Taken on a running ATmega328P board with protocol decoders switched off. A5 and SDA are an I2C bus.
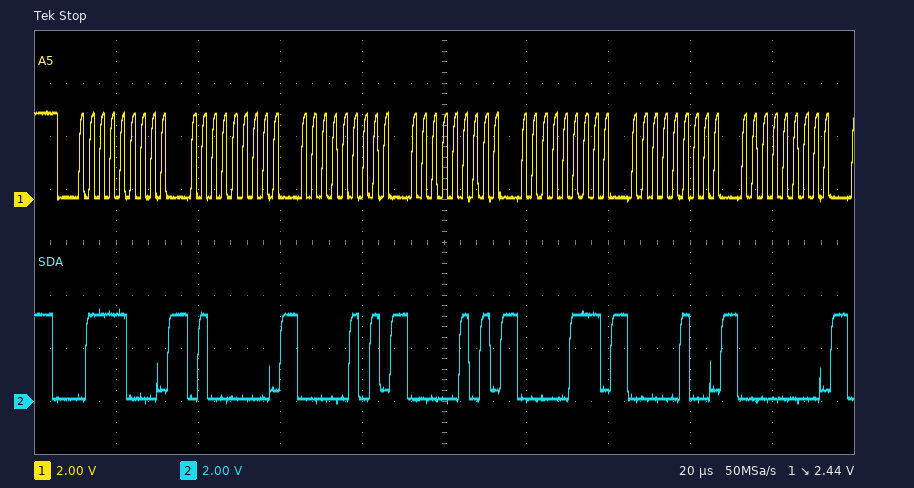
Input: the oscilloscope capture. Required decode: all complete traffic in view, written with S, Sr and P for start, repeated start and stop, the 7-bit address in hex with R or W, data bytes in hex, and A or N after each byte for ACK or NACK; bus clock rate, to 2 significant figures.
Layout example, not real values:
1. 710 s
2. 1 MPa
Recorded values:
1. S 3CW A 40 A 05 A 05 A 07 A 04 A 00 A
2. 400 kHz
